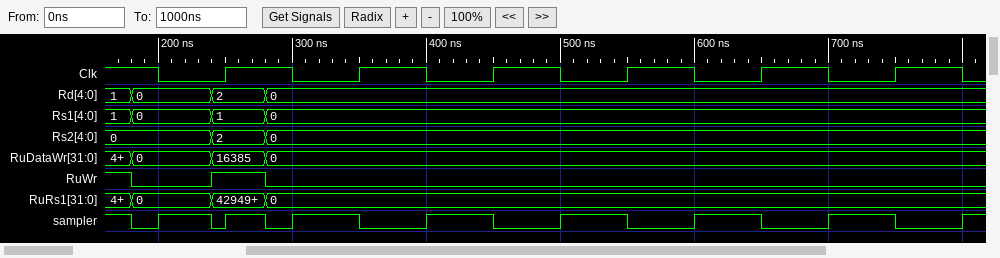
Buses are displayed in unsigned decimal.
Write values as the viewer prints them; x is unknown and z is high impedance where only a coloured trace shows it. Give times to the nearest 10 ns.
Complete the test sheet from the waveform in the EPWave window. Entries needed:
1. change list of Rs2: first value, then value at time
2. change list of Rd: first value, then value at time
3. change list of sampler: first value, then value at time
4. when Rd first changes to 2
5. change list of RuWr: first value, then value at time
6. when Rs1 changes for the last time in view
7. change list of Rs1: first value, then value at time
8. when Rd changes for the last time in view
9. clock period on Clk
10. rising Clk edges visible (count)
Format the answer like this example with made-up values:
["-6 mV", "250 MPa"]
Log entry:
["0, 2 at 240 ns, 0 at 280 ns", "1, 0 at 180 ns, 2 at 240 ns, 0 at 280 ns", "1, 0 at 180 ns, 1 at 200 ns, 0 at 240 ns, 1 at 250 ns, 0 at 280 ns, 1 at 300 ns, 0 at 350 ns, 1 at 400 ns, 0 at 450 ns, 1 at 500 ns, 0 at 550 ns, 1 at 600 ns, 0 at 650 ns, 1 at 700 ns, 0 at 750 ns, 1 at 800 ns", "240 ns", "1, 0 at 180 ns, 1 at 240 ns, 0 at 280 ns", "280 ns", "1, 0 at 180 ns, 1 at 240 ns, 0 at 280 ns", "280 ns", "100 ns", "6"]
